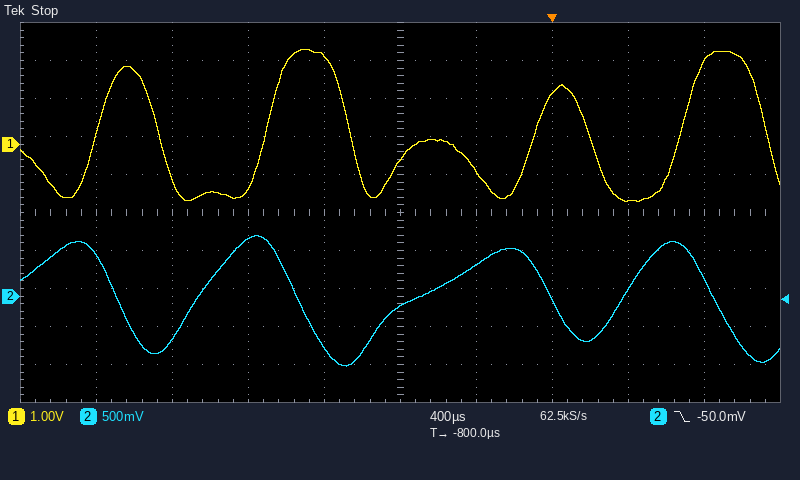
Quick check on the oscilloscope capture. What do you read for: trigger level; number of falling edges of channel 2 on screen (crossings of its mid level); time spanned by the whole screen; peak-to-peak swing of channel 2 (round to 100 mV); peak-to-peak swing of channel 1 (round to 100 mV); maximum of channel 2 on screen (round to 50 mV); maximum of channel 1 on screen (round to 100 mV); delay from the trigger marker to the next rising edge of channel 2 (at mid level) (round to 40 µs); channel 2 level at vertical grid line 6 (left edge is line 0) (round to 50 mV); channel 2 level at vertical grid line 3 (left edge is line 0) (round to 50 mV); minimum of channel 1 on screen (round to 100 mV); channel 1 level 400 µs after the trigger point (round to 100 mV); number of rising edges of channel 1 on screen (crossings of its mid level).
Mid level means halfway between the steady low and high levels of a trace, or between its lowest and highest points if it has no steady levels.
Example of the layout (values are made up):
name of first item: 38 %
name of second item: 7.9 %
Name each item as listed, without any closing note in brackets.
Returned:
trigger level: -50.0 mV
number of falling edges of channel 2 on screen: 4
time spanned by the whole screen: 4 ms
peak-to-peak swing of channel 2: 1.70 V
peak-to-peak swing of channel 1: 4.0 V
maximum of channel 2 on screen: 800 mV
maximum of channel 1 on screen: 2.5 V
delay from the trigger marker to the next rising edge of channel 2 (at mid level): 360 µs
channel 2 level at vertical grid line 6 (left edge is line 0): 400 mV
channel 2 level at vertical grid line 3 (left edge is line 0): 750 mV
minimum of channel 1 on screen: -1.5 V
channel 1 level 400 µs after the trigger point: -1.5 V
number of rising edges of channel 1 on screen: 4
